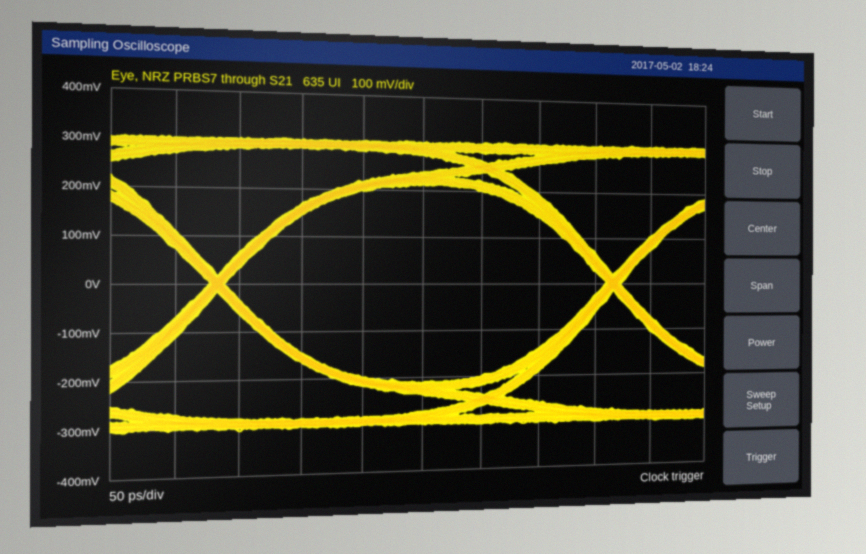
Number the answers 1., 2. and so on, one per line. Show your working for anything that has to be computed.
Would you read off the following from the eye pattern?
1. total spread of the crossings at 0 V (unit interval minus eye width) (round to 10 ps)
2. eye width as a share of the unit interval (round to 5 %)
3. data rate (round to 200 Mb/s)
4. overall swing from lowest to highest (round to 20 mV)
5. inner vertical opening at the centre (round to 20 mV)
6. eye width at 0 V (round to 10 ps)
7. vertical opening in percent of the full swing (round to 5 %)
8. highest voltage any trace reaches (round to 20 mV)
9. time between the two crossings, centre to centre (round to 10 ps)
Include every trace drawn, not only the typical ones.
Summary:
1. 10 ps
2. 320 ps / 330 ps ≈ 97.0 %, so 95 % to the nearest 5 %
3. 3.0 Gb/s
4. 620 mV
5. 420 mV
6. 320 ps
7. 420 mV / 620 mV ≈ 67.7 %, so 70 % to the nearest 5 %
8. 300 mV
9. 330 ps
